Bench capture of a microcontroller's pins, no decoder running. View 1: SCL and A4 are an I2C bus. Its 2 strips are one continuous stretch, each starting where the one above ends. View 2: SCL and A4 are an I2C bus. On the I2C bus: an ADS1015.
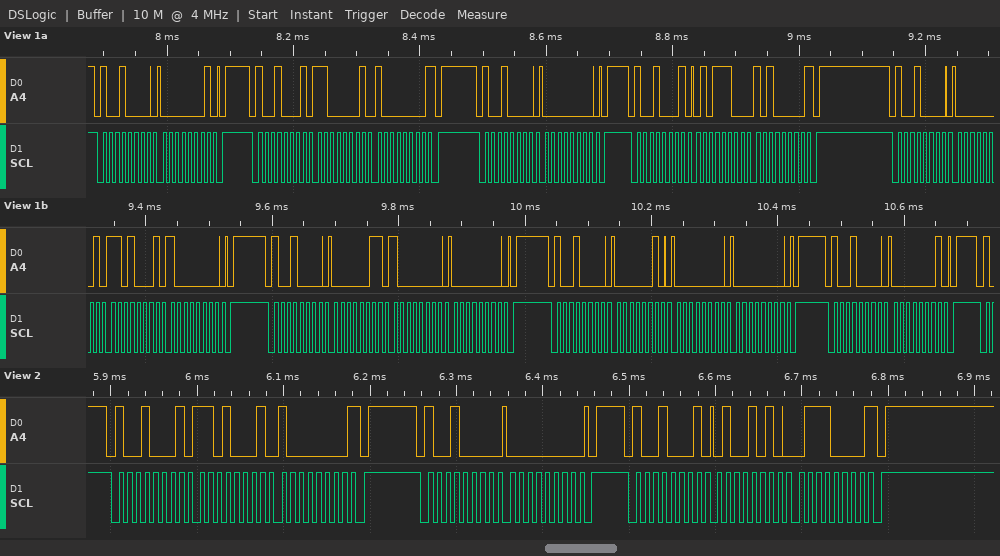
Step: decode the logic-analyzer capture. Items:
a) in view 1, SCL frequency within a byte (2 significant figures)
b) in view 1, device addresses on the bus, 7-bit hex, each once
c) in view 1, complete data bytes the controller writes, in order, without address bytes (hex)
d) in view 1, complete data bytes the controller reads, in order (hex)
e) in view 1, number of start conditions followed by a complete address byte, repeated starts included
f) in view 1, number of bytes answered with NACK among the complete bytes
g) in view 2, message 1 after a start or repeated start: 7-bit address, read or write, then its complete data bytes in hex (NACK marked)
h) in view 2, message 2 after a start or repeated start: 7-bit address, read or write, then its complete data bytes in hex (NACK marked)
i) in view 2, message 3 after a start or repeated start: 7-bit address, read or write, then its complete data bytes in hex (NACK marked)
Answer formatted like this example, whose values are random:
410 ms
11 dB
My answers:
100 kHz
0x48
01 00 01 D1 80 03 80 00 02 00 00 01
C1 80 5C A0
8
2
0x48 read: D1 80 NACK
0x48 write: 00
0x48 read: 4A 70 NACK
